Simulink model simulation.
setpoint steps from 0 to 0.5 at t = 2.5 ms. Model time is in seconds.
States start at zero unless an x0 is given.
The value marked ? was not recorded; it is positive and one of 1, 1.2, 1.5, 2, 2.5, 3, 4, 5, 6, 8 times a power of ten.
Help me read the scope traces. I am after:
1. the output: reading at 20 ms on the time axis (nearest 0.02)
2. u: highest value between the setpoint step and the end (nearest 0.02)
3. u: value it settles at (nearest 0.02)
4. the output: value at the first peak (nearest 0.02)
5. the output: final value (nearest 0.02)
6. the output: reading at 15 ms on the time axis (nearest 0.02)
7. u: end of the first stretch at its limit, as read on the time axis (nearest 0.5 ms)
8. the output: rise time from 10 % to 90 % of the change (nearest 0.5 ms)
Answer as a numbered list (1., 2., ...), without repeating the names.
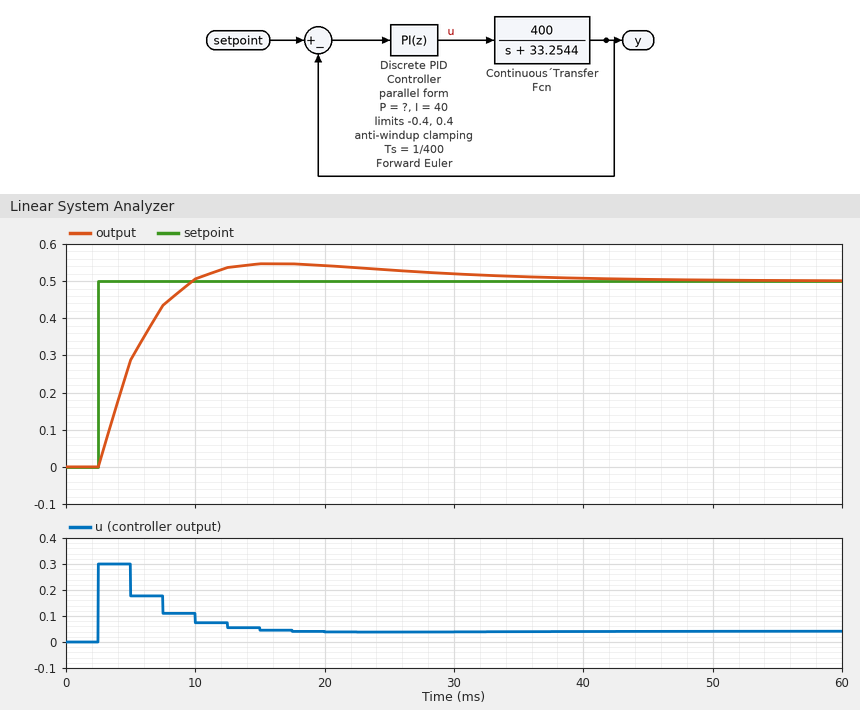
1. 0.54
2. 0.30
3. 0.04
4. 0.54
5. 0.50
6. 0.54
7. 5.0 ms
8. 5.0 ms
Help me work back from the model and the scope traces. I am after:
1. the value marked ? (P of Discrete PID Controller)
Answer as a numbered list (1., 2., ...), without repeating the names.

1. 0.6
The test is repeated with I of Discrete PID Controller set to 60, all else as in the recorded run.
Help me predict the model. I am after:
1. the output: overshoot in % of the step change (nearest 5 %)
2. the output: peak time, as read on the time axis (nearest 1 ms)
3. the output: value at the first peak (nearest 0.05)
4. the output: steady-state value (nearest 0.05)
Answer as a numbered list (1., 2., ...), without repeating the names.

1. 20 %
2. 15 ms
3. 0.60
4. 0.50
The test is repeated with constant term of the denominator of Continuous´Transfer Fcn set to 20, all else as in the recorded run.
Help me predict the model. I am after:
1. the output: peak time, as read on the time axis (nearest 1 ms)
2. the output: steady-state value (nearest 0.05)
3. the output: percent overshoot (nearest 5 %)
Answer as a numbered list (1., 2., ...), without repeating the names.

1. 15 ms
2. 0.50
3. 15 %
